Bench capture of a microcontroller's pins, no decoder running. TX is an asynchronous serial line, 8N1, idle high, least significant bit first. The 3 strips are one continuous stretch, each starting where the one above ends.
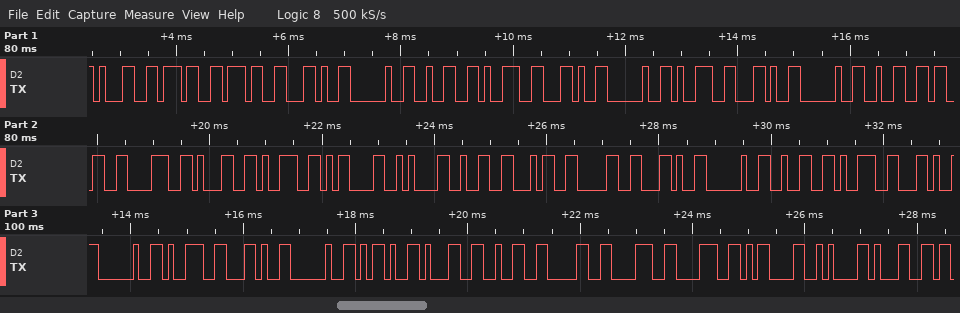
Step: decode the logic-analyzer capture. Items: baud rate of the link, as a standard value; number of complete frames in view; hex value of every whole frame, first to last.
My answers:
9600 baud
40
0x31 0x37 0x37 0x2C 0x20 0x32 0x39 0x2C 0x20 0x39 0x2C 0x20 0x32 0x33 0x38 0x31 0x39 0x0D 0x0A 0x32 0x34 0x30 0x2C 0x20 0x32 0x39 0x2C 0x20 0x39 0x2C 0x20 0x2D 0x31 0x32 0x30 0x38 0x38 0x0D 0x0A 0x31
